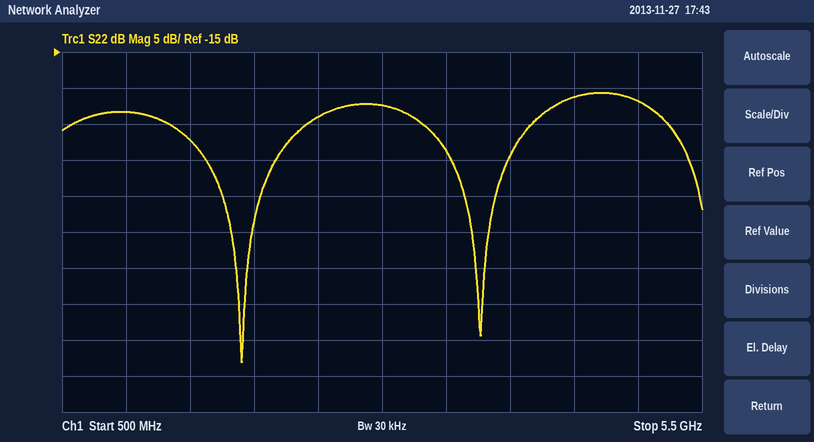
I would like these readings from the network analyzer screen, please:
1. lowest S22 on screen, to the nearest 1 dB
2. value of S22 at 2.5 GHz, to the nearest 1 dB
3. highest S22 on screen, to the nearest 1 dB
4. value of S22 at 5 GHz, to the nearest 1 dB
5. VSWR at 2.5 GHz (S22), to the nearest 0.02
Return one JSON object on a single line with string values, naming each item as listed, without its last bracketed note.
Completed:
{"lowest S22 on screen, to the nearest 1 dB": "-58 dB", "value of S22 at 2.5 GHz, to the nearest 1 dB": "-24 dB", "highest S22 on screen, to the nearest 1 dB": "-21 dB", "value of S22 at 5 GHz, to the nearest 1 dB": "-22 dB", "VSWR at 2.5 GHz (S22), to the nearest 0.02": "1.14"}
